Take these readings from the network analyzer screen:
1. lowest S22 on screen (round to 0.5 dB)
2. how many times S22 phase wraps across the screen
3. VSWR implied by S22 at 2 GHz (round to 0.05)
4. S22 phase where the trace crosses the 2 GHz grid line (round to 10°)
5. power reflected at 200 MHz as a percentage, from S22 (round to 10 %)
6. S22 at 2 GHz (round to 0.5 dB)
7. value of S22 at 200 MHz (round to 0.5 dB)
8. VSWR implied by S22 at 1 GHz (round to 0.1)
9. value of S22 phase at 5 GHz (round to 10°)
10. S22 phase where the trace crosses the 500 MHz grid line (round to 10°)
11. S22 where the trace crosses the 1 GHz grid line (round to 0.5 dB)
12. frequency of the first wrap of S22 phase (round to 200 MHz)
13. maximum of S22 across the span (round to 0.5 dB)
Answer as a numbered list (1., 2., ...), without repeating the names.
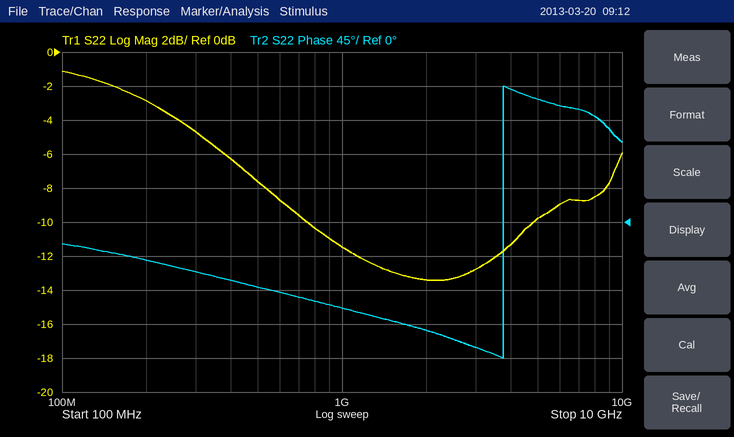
1. -13.5 dB
2. 1
3. 1.55
4. -140°
5. 50 %
6. -13.5 dB
7. -3.0 dB
8. 1.7
9. 160°
10. -90°
11. -11.5 dB
12. 3.8 GHz
13. -1.0 dB
